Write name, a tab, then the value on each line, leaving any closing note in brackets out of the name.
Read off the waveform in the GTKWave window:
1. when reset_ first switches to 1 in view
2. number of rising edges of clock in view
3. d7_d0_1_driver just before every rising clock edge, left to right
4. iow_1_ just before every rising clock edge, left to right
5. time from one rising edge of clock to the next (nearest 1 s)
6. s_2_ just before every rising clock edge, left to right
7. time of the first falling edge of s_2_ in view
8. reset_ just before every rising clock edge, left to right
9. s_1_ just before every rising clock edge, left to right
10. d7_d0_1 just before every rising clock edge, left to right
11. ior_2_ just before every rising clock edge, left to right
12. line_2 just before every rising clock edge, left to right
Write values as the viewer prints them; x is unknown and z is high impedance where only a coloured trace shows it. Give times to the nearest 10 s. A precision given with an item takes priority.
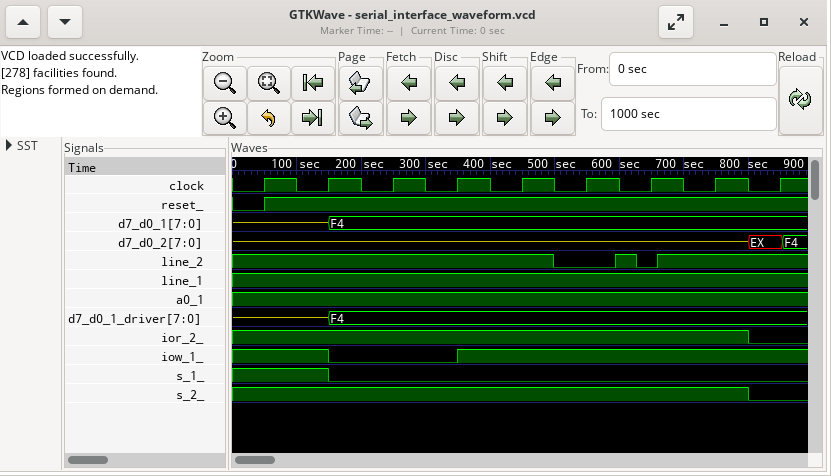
when reset_ first switches to 1 in view	50 s
number of rising edges of clock in view	9
d7_d0_1_driver just before every rising clock edge, left to right	z, z, F4, F4, F4, F4, F4, F4, F4
iow_1_ just before every rising clock edge, left to right	1 1 0 0 1 1 1 1 1
time from one rising edge of clock to the next	100 s
s_2_ just before every rising clock edge, left to right	1 1 1 1 1 1 1 1 0
time of the first falling edge of s_2_ in view	800 s
reset_ just before every rising clock edge, left to right	0 1 1 1 1 1 1 1 1
s_1_ just before every rising clock edge, left to right	1 1 0 0 0 0 0 0 0
d7_d0_1 just before every rising clock edge, left to right	z, z, F4, F4, F4, F4, F4, F4, F4
ior_2_ just before every rising clock edge, left to right	1 1 1 1 1 1 1 1 0
line_2 just before every rising clock edge, left to right	1 1 1 1 1 0 0 1 1
